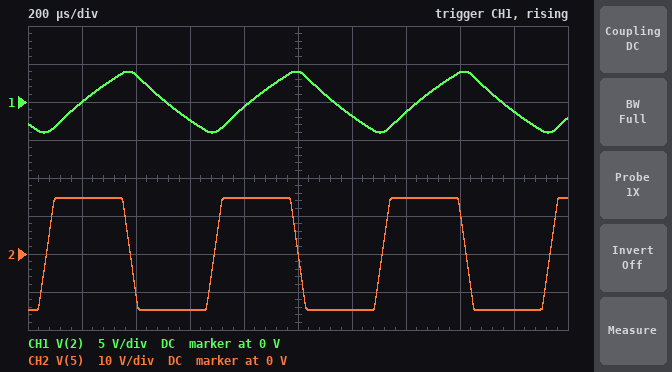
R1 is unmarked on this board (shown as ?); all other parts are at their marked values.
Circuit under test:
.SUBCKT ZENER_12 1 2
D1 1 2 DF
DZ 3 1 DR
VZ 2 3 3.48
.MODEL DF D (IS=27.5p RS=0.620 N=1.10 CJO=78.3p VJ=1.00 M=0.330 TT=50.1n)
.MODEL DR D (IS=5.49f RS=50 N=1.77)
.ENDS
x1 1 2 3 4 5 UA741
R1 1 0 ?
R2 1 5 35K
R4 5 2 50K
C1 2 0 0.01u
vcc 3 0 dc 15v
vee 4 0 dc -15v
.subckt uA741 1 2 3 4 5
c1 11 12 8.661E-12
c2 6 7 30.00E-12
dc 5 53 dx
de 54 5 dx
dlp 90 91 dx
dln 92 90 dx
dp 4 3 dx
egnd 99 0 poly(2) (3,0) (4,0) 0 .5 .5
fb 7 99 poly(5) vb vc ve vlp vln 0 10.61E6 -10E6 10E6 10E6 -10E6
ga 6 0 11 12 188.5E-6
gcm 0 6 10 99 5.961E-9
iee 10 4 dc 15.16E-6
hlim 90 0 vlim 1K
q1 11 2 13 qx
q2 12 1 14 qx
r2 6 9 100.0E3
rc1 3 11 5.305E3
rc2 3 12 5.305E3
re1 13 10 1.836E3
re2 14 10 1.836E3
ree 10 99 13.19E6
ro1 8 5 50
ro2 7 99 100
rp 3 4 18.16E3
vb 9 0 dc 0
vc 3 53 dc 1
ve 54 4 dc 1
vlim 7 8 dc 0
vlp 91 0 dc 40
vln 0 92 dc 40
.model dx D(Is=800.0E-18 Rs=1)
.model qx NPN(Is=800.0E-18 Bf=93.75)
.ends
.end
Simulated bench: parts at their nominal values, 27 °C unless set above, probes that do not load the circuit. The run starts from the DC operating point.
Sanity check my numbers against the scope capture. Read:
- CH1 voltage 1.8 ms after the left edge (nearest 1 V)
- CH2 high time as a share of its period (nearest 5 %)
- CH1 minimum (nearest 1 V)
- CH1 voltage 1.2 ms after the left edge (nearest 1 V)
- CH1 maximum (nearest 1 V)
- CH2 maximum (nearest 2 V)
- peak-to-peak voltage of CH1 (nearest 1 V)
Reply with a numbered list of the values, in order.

1. -1 V
2. 50 %
3. -4 V
4. -2 V
5. 4 V
6. 14 V
7. 8 V
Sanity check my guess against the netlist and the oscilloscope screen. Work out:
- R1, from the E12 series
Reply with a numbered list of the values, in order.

1. 12 kΩ
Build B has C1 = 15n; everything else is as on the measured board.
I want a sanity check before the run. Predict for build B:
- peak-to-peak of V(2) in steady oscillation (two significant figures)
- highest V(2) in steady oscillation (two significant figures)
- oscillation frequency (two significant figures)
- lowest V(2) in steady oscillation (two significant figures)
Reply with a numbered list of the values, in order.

1. 7.8 V
2. 3.9 V
3. 1.1 kHz
4. -3.9 V
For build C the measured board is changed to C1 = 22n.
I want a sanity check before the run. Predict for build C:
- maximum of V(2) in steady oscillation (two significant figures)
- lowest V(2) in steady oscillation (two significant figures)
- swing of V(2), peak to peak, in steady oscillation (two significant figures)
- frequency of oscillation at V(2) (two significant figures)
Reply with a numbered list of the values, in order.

1. 3.9 V
2. -3.9 V
3. 7.7 V
4. 800 Hz
